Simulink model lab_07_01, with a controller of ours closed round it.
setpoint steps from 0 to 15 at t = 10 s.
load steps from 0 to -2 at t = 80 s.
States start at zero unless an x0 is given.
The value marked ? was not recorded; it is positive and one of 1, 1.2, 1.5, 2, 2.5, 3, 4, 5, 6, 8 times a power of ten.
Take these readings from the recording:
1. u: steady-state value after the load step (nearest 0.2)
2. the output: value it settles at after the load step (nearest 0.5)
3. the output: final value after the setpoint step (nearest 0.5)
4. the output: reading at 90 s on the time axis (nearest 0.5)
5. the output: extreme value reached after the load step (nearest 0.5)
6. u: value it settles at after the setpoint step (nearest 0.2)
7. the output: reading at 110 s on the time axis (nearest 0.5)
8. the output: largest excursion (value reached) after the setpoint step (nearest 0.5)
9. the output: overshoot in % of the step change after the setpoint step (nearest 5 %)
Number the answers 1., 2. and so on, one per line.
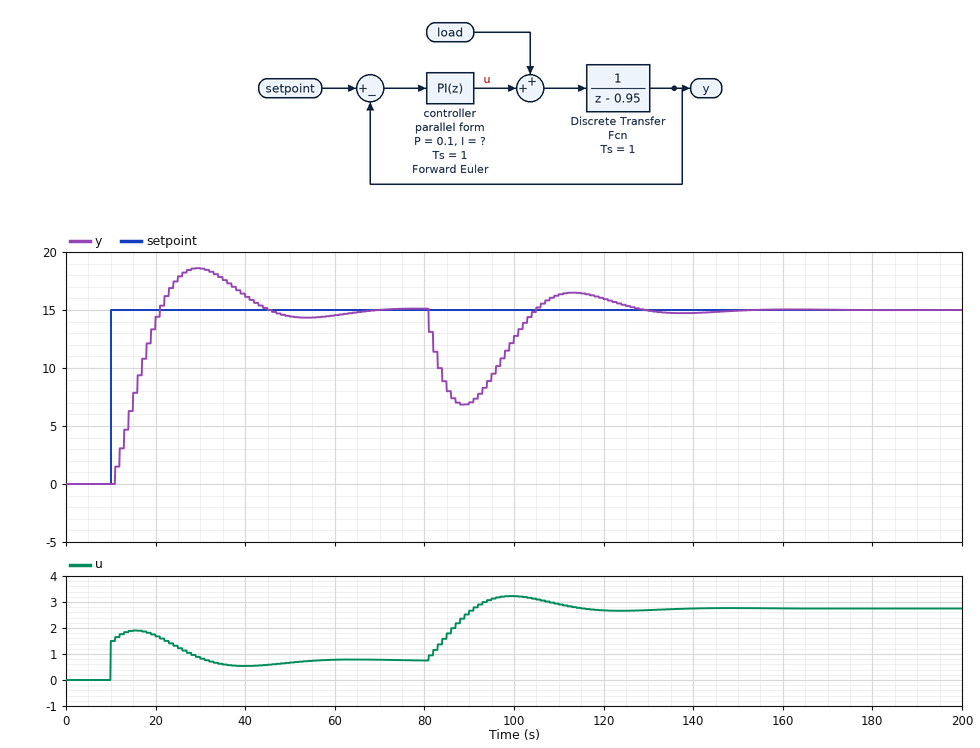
1. 2.8
2. 15.0
3. 15.0
4. 7.0
5. 7.0
6. 0.8
7. 16.5
8. 18.5
9. 25 %
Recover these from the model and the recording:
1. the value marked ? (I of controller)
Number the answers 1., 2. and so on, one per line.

1. 0.02
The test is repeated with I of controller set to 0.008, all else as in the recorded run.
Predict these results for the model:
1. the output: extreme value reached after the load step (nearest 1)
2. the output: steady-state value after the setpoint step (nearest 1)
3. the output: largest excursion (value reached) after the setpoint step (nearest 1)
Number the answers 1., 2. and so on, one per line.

1. 5
2. 15
3. 16
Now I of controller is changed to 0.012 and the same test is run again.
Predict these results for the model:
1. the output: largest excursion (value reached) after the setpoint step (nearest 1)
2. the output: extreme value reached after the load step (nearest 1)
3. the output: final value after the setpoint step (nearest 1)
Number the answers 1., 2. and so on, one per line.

1. 17
2. 6
3. 15
